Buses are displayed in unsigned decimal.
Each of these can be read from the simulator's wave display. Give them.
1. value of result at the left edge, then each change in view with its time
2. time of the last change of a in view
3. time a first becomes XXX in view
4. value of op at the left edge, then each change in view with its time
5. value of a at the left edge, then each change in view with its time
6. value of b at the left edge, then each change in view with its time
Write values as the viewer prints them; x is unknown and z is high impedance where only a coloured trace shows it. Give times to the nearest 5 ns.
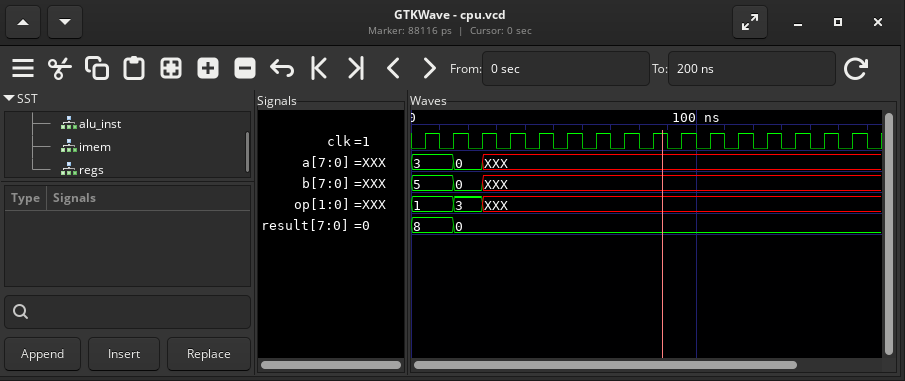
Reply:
8, 0 at 15 ns
25 ns
25 ns
1, 3 at 15 ns, XXX at 25 ns
3, 0 at 15 ns, XXX at 25 ns
5, 0 at 15 ns, XXX at 25 ns
